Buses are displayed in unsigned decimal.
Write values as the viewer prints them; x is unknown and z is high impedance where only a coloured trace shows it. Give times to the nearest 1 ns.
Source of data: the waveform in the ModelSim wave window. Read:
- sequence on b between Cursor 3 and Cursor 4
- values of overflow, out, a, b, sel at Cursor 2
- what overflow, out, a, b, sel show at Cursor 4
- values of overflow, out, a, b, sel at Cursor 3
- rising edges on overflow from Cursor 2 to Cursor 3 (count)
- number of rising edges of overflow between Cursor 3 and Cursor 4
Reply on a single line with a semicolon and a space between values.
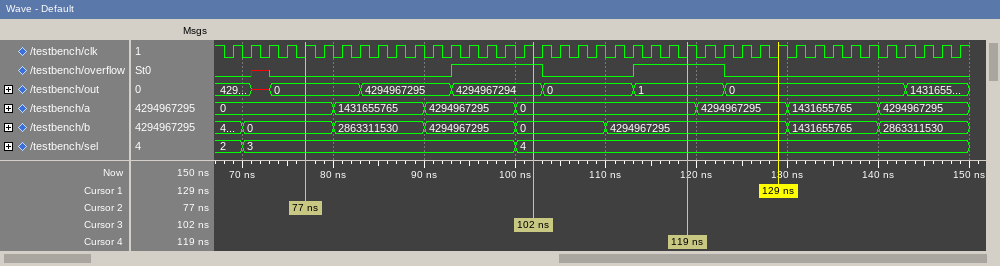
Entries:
0, 4294967295; overflow=0, out=0, a=0, b=0, sel=3; overflow=1, out=1, a=0, b=4294967295, sel=4; overflow=1, out=4294967294, a=0, b=0, sel=4; 1; 1
